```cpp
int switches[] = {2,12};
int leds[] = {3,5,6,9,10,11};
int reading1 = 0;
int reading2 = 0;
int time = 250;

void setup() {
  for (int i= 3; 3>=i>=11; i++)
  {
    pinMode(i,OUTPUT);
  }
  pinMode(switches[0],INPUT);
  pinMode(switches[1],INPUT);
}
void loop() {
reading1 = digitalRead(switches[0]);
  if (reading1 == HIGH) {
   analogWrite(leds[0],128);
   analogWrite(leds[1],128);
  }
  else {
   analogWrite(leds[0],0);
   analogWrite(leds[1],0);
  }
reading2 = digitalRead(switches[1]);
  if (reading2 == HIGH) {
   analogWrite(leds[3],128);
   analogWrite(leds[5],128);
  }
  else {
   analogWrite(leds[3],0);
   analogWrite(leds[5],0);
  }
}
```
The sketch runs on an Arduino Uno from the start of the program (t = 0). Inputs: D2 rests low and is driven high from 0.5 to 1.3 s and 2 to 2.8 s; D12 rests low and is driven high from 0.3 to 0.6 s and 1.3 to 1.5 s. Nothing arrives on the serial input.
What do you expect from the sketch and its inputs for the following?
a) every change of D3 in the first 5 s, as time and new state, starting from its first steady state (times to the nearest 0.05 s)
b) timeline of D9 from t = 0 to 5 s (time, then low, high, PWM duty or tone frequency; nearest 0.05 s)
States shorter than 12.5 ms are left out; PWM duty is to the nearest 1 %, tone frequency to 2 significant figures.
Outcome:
0 s low; 0.5 s PWM 50 %; 1.3 s low; 2 s PWM 50 %; 2.8 s low
0 s low; 0.3 s PWM 50 %; 0.6 s low; 1.3 s PWM 50 %; 1.5 s low
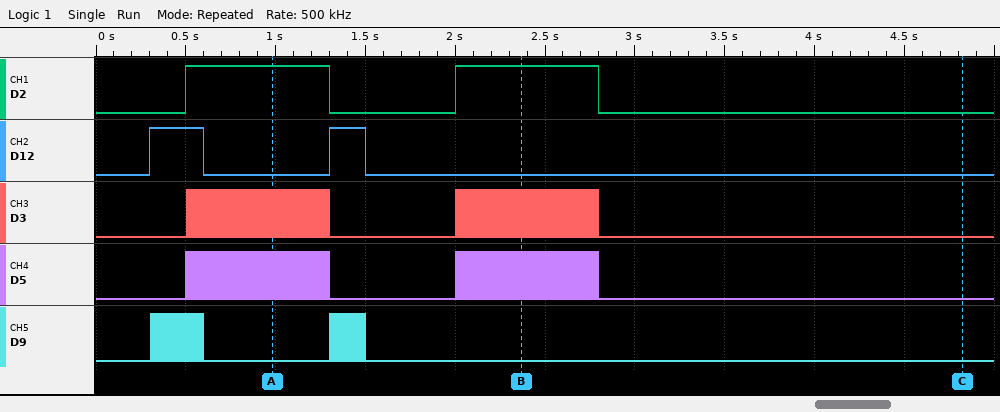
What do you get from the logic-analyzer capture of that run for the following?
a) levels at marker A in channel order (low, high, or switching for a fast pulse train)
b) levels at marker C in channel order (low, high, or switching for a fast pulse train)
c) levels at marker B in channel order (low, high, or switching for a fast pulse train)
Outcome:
D2 high, D12 low, D3 switching, D5 switching, D9 low
D2 low, D12 low, D3 low, D5 low, D9 low
D2 high, D12 low, D3 switching, D5 switching, D9 low
